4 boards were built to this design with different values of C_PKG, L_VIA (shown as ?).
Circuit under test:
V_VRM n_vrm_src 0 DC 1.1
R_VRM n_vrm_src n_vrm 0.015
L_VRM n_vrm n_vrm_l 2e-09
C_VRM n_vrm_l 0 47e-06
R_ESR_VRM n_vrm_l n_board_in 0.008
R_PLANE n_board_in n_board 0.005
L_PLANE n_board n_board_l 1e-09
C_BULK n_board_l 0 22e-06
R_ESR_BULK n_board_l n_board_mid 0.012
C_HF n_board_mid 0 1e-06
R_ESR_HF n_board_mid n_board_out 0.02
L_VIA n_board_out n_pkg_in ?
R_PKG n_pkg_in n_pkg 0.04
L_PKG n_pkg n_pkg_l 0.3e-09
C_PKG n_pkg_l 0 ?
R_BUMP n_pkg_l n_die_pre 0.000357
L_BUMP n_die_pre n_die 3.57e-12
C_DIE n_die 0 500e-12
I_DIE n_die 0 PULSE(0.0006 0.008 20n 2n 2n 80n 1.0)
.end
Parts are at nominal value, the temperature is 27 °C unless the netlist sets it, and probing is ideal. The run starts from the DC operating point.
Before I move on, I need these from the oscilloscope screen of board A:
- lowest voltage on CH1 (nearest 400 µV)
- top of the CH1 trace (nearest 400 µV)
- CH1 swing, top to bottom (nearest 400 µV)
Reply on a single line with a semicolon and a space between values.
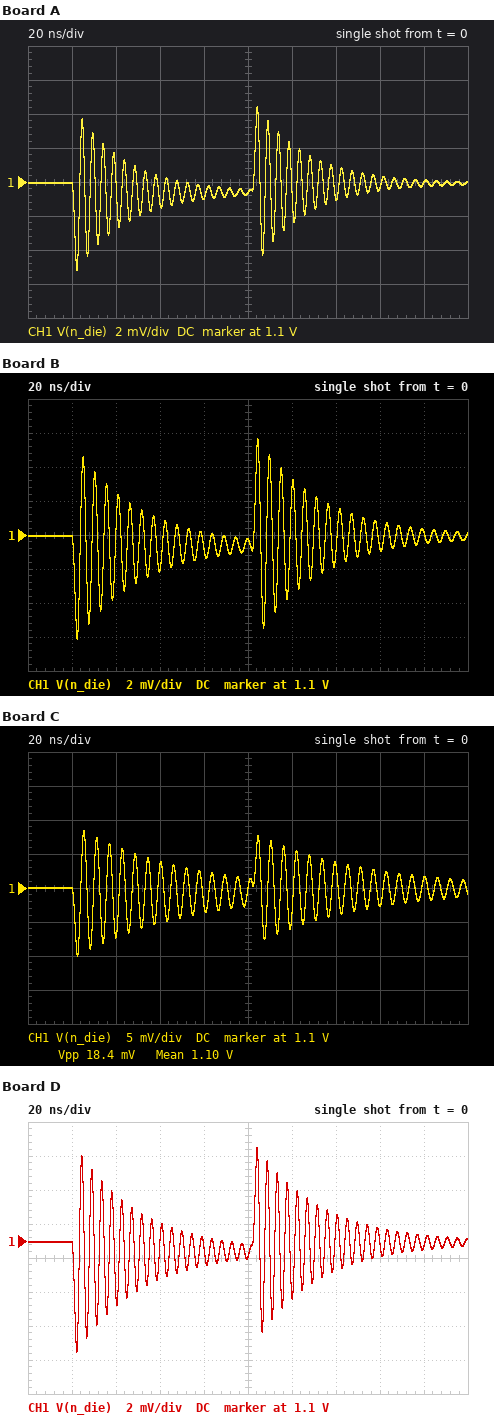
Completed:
1.0948 V; 1.1044 V; 9.6 mV
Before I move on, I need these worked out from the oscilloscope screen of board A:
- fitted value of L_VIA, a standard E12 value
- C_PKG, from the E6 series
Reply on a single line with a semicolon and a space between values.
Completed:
390 pH; 330 pF
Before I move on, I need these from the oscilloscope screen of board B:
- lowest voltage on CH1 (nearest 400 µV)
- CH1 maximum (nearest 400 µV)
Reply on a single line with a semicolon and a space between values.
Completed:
1.0940 V; 1.1056 V
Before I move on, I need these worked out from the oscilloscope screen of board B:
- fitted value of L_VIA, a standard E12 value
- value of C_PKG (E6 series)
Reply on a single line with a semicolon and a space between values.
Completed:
560 pH; 330 pF
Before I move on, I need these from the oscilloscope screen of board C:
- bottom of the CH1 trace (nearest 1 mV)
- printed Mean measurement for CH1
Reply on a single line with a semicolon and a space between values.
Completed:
1.090 V; 1.10 V
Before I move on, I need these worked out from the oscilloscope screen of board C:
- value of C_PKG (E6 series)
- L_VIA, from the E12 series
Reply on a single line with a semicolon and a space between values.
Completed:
68 pF; 1.2 nH
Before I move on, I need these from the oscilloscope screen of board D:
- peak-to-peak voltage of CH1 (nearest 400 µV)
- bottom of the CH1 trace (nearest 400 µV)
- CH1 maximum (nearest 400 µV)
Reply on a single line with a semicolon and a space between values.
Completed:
12.0 mV; 1.0936 V; 1.1056 V
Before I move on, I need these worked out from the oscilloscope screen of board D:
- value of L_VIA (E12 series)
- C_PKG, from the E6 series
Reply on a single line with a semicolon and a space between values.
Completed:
560 pH; 100 pF
